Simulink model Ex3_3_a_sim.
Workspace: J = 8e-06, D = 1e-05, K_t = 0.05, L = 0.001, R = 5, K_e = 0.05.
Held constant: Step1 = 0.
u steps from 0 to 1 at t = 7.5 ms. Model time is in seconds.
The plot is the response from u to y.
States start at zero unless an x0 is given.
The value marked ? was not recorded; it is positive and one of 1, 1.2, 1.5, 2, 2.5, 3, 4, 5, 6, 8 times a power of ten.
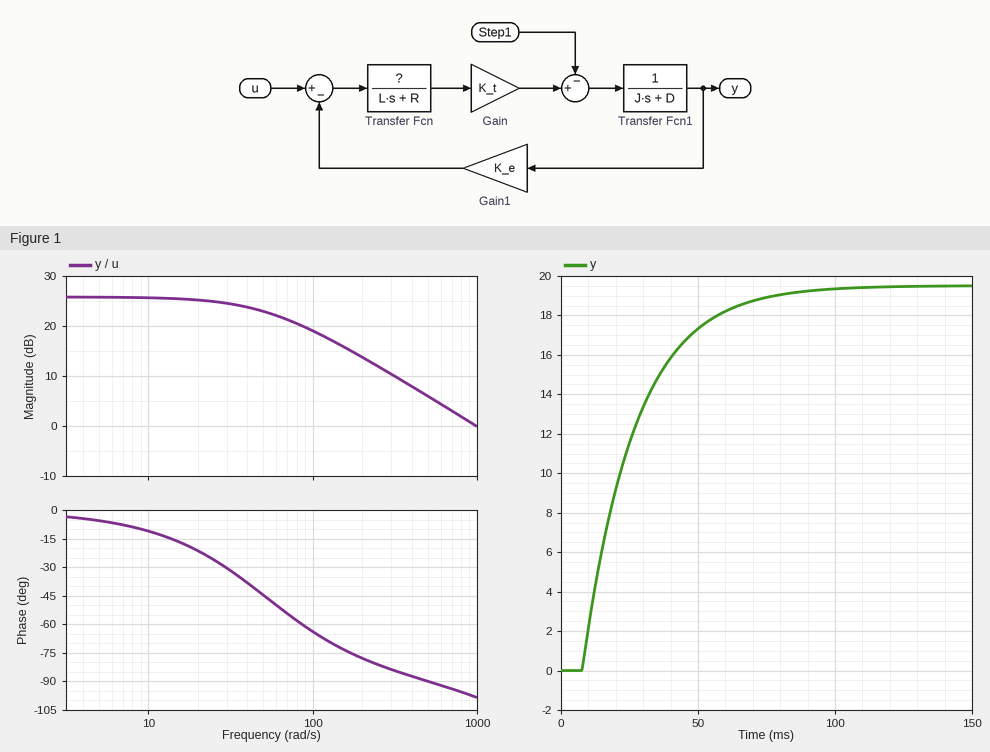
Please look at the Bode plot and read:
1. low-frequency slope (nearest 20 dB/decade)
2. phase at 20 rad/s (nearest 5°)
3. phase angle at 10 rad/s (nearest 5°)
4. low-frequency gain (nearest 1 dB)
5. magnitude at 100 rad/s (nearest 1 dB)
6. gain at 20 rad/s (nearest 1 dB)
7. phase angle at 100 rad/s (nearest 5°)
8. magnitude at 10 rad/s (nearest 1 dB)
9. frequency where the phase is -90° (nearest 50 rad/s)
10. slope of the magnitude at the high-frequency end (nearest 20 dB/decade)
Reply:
0 dB/decade
-20°
-10°
26 dB
19 dB
25 dB
-65°
26 dB
500 rad/s
-20 dB/decade
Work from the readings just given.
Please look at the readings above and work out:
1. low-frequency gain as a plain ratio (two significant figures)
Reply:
20
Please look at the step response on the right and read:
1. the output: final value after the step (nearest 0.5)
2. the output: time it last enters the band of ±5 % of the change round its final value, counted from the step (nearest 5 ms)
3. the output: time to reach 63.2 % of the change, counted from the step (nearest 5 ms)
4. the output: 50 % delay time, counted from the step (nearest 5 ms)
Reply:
19.5
60 ms
20 ms
15 ms
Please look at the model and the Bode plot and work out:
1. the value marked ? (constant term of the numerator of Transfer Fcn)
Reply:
0.8
